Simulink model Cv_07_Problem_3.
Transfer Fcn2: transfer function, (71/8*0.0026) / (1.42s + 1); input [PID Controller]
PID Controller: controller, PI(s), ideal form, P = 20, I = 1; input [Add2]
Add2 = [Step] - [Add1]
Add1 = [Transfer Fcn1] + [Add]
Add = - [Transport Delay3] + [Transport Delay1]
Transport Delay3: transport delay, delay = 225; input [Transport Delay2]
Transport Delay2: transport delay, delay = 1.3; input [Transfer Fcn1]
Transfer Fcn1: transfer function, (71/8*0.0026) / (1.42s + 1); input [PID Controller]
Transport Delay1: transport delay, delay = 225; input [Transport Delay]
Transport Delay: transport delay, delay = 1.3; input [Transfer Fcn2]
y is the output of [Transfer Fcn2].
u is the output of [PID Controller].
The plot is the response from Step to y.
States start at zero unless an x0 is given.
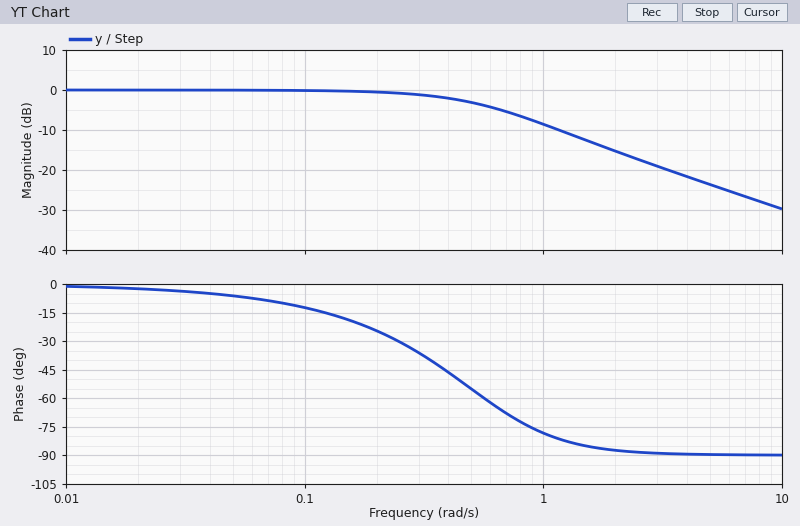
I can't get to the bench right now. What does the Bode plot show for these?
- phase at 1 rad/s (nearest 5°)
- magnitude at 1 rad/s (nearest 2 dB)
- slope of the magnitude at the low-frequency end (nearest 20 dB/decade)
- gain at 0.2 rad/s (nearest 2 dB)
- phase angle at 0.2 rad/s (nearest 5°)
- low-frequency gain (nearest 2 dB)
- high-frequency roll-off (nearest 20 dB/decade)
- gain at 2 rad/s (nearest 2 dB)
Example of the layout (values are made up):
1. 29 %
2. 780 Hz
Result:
1. -80°
2. -8 dB
3. 0 dB/decade
4. 0 dB
5. -25°
6. 0 dB
7. -20 dB/decade
8. -16 dB
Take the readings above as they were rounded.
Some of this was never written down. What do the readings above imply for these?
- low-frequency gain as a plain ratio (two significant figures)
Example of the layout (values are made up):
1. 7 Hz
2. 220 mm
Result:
1. 1.0
